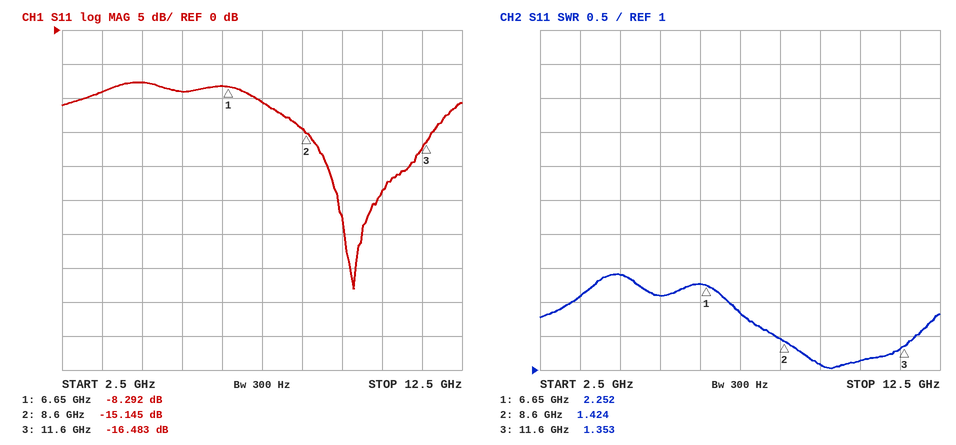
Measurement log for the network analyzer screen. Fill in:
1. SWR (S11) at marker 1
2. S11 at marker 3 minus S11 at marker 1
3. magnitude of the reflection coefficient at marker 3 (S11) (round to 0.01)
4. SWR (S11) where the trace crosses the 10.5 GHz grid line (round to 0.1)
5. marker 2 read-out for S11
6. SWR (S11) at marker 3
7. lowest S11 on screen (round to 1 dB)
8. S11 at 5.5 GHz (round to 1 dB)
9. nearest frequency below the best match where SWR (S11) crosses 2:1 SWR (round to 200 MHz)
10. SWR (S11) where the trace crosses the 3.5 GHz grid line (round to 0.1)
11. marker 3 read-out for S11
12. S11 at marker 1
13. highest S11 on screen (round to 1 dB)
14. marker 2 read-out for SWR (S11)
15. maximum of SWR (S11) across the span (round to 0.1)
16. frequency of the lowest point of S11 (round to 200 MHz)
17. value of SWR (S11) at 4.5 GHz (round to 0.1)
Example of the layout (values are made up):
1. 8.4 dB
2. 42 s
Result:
1. 2.252
2. -8.191 dB
3. 0.15
4. 1.1
5. -15.145 dB
6. 1.353
7. -38 dB
8. -9 dB
9. 7.2 GHz
10. 2.1
11. -16.483 dB
12. -8.292 dB
13. -8 dB
14. 1.424
15. 2.4
16. 9.8 GHz
17. 2.4
